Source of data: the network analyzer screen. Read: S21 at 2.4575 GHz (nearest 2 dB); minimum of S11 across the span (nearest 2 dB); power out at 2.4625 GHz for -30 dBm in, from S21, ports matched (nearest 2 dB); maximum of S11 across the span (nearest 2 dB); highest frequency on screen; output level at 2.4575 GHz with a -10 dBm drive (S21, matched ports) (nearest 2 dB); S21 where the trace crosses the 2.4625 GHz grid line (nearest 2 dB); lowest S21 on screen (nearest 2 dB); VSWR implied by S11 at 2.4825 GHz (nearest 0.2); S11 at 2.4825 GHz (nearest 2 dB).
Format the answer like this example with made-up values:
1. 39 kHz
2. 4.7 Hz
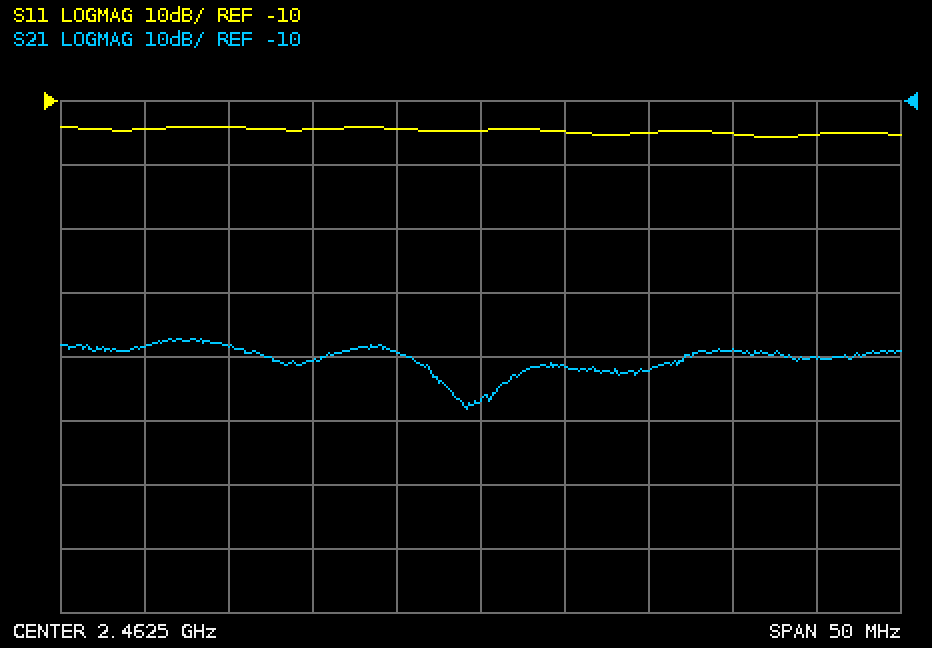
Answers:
1. -50 dB
2. -16 dB
3. -86 dBm
4. -14 dB
5. 2.4875 GHz
6. -60 dBm
7. -56 dB
8. -58 dB
9. 1.4
10. -16 dB
